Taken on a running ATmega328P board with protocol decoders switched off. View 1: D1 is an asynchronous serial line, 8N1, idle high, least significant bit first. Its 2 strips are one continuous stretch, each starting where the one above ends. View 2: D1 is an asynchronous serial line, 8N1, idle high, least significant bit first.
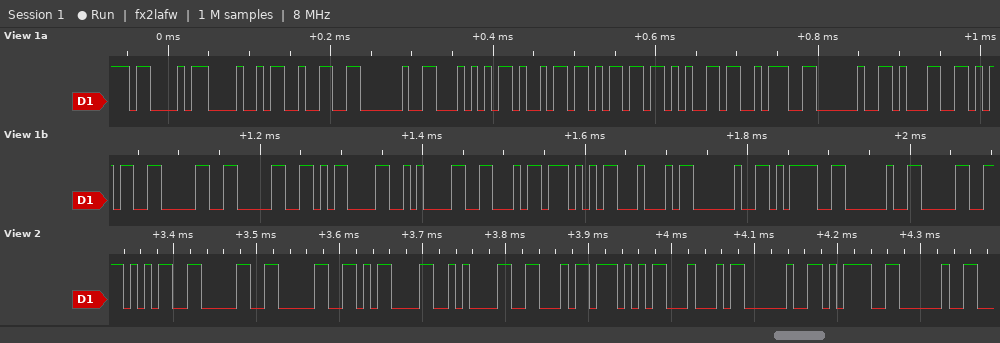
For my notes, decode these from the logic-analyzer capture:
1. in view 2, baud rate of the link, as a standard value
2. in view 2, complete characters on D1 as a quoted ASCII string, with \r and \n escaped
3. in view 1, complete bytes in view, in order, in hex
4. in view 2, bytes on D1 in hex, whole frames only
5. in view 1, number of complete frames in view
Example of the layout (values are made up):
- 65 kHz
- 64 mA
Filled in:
- 115200 baud
- "500\r\nFWD = "
- 43 48 32 20 54 69 6D 65 3A 20 31 35 30 30 0D 0A 46 57 44 20 3D 20 30
- 0x35 0x30 0x30 0x0D 0x0A 0x46 0x57 0x44 0x20 0x3D 0x20
- 23
